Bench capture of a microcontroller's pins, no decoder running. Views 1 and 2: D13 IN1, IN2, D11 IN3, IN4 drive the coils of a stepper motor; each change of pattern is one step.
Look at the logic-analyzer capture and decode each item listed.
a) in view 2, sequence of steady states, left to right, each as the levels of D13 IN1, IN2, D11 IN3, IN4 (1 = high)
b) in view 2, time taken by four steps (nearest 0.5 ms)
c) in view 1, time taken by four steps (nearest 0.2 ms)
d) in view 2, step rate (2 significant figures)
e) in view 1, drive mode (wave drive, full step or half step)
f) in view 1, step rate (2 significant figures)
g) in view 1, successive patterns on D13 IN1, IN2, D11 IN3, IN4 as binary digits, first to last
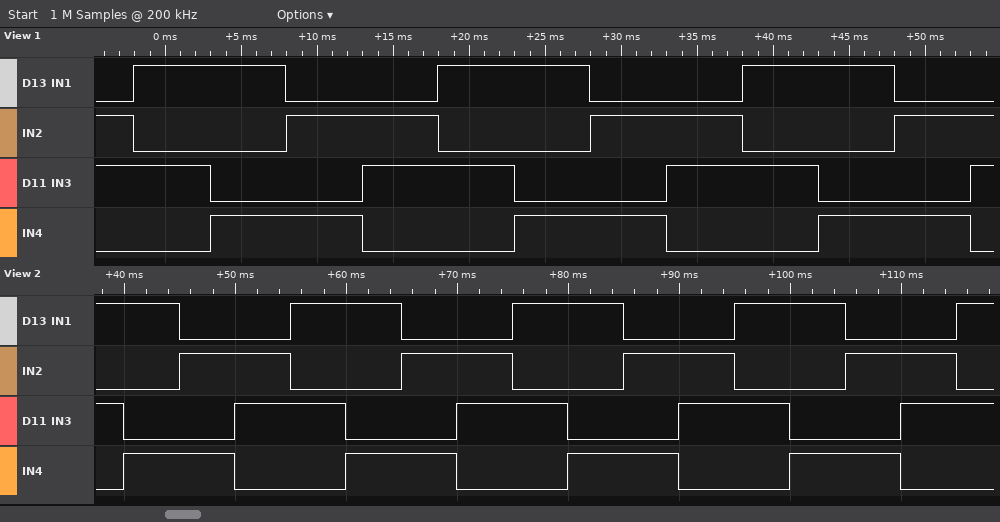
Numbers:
1010 1001 0101 0110 1010 1001 0101 0110 1010 1001 0101 0110 1010 1001 0101 0110 1010
20.0 ms
20.0 ms
200 steps/s
full step
200 steps/s
0110 1010 1001 0101 0110 1010 1001 0101 0110 1010 1001 0101 0110
